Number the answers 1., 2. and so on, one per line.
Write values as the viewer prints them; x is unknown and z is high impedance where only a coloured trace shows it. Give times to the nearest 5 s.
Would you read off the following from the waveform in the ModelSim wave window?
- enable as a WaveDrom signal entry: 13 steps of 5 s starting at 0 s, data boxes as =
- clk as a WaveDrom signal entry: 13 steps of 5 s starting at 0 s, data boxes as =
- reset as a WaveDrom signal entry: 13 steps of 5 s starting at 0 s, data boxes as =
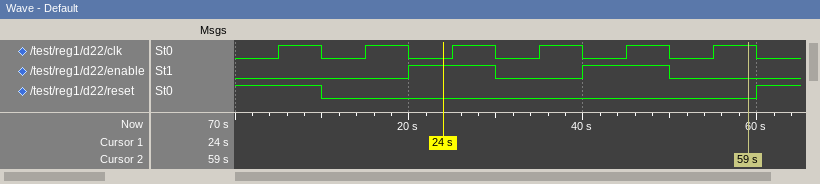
1. {name: 'enable', wave: '0...1.0.1.0..'}
2. {name: 'clk', wave: '0101010101010'}
3. {name: 'reset', wave: '1.0.........1'}
